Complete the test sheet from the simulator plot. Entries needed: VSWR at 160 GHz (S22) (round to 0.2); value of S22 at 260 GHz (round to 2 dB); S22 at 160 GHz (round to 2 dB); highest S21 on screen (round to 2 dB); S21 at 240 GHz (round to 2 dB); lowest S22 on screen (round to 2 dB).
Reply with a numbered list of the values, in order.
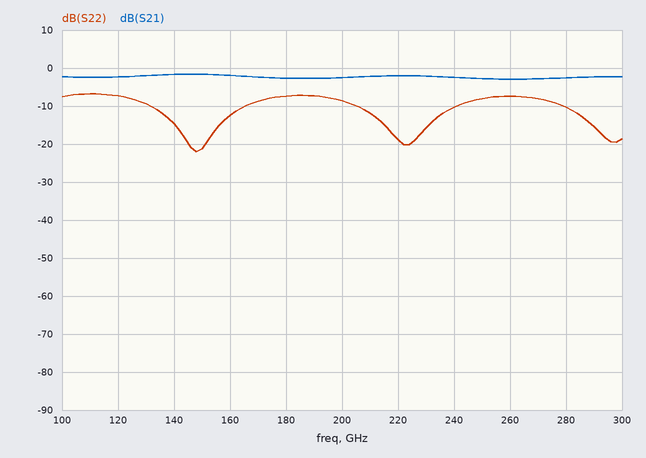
1. 1.6
2. -8 dB
3. -12 dB
4. -2 dB
5. -2 dB
6. -22 dB
